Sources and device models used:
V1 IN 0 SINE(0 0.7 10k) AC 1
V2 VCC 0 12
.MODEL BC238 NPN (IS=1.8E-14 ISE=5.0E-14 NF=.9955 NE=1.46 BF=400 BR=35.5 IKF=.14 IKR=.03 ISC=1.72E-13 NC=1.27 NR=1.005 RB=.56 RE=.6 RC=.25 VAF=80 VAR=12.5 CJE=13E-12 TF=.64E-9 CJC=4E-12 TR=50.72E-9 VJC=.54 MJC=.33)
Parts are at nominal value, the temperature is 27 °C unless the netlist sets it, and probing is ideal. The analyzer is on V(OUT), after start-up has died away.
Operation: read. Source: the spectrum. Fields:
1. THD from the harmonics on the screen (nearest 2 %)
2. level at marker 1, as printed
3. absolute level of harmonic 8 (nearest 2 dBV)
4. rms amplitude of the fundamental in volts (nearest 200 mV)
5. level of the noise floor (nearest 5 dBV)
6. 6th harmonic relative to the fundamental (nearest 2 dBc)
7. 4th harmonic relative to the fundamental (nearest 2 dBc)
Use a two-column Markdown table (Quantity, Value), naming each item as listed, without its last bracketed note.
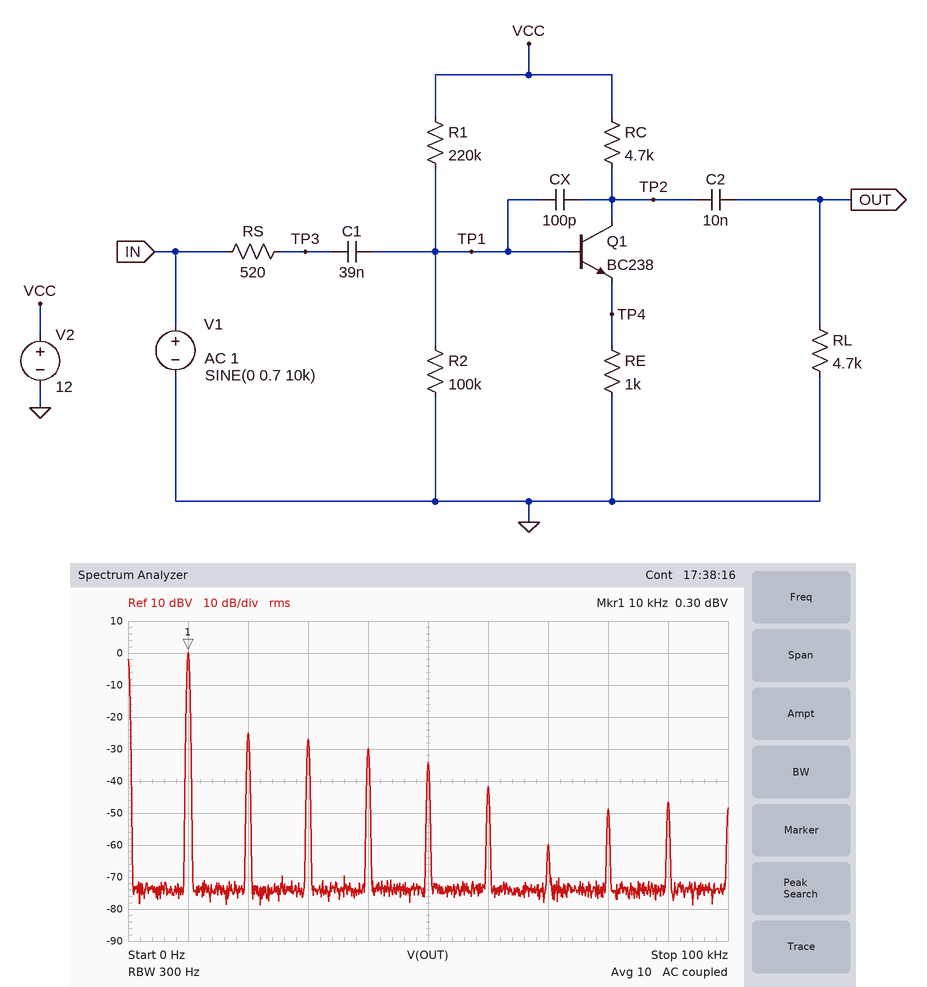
| Quantity | Value |
|---|---|
| THD from the harmonics on the screen | 8 % |
| level at marker 1, as printed | 0.30 dBV |
| absolute level of harmonic 8 | -48 dBV |
| rms amplitude of the fundamental in volts | 1.0 V |
| level of the noise floor | -75 dBV |
| 6th harmonic relative to the fundamental | -42 dBc |
| 4th harmonic relative to the fundamental | -30 dBc |
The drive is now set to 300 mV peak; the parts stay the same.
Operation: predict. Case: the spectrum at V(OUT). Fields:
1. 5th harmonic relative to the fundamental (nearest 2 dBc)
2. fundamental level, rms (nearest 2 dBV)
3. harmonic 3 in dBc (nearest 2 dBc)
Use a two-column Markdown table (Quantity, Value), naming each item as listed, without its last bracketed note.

| Quantity | Value |
|---|---|
| 5th harmonic relative to the fundamental | -38 dBc |
| fundamental level, rms | -8 dBV |
| harmonic 3 in dBc | -24 dBc |
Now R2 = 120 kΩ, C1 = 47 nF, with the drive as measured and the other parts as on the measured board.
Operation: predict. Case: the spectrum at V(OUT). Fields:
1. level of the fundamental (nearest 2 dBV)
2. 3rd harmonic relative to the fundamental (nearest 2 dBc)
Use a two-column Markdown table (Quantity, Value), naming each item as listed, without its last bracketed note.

| Quantity | Value |
|---|---|
| level of the fundamental | 0 dBV |
| 3rd harmonic relative to the fundamental | -26 dBc |
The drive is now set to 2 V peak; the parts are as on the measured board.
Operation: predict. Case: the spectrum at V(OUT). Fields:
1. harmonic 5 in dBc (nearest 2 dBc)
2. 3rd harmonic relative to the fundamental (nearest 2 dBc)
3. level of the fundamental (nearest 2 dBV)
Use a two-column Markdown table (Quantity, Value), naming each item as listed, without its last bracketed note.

| Quantity | Value |
|---|---|
| harmonic 5 in dBc | -36 dBc |
| 3rd harmonic relative to the fundamental | -18 dBc |
| level of the fundamental | 8 dBV |
